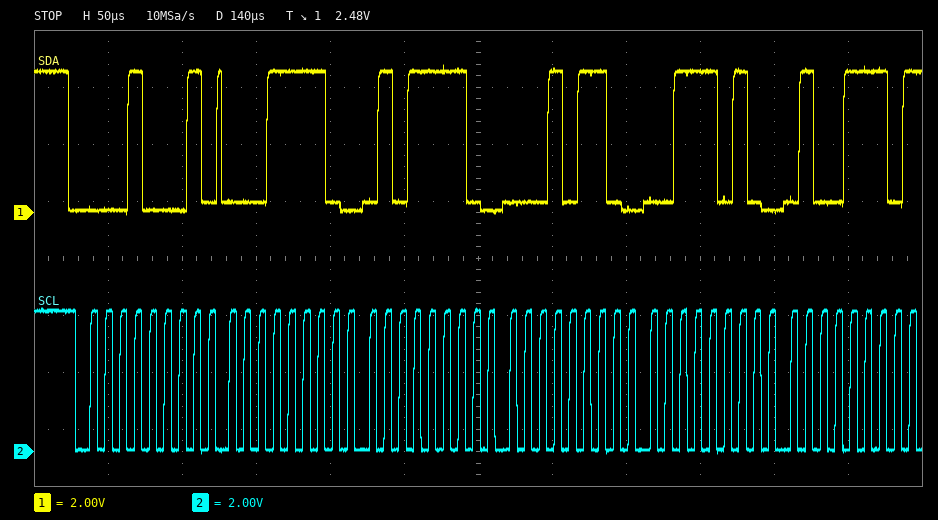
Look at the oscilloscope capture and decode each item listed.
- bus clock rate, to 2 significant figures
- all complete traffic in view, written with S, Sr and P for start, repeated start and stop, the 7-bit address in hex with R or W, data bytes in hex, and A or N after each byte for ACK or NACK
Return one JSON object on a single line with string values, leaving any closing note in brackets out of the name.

{"bus clock rate, to 2 significant figures": "100 kHz", "all complete traffic in view, written with S, Sr and P for start, repeated start and stop, the 7-bit address in hex with R or W, data bytes in hex, and A or N after each byte for ACK or NACK": "S 08R A 1E A 5E A 16 A 3A A 4E N"}
